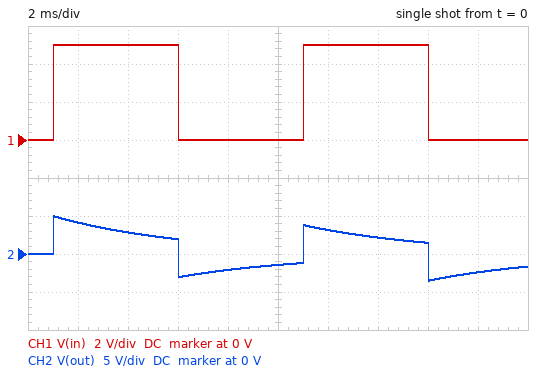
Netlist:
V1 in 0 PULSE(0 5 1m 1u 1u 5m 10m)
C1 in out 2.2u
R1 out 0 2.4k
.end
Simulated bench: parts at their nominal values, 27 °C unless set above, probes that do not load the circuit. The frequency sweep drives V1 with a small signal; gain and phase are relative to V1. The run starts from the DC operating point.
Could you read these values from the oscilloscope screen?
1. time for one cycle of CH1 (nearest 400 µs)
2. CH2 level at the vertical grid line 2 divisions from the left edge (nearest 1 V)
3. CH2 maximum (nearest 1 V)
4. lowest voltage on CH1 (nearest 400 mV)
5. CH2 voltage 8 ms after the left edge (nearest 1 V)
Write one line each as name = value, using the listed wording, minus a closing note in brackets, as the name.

time for one cycle of CH1 = 10.0 ms
CH2 level at the vertical grid line 2 divisions from the left edge = 3 V
CH2 maximum = 5 V
lowest voltage on CH1 = 0 V
CH2 voltage 8 ms after the left edge = -2 V
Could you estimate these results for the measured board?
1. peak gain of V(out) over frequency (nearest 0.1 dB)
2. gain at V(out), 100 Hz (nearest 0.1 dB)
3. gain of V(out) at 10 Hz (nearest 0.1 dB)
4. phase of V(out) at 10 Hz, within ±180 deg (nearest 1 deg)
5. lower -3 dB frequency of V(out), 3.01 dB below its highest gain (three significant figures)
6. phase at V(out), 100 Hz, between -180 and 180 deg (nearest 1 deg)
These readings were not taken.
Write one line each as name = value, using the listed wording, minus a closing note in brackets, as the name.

peak gain of V(out) over frequency = 0 dB
gain at V(out), 100 Hz = -0.4 dB
gain of V(out) at 10 Hz = -10.0 dB
phase of V(out) at 10 Hz, within ±180 deg = 72 deg
lower -3 dB frequency of V(out), 3.01 dB below its highest gain = 30.1 Hz
phase at V(out), 100 Hz, between -180 and 180 deg = 17 deg
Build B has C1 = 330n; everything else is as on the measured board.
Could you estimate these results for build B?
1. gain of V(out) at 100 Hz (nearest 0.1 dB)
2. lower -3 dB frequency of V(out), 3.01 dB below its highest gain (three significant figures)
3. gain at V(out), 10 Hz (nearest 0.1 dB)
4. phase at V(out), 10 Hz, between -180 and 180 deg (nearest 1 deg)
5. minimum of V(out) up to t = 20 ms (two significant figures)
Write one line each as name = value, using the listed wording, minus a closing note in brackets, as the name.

gain of V(out) at 100 Hz = -7.0 dB
lower -3 dB frequency of V(out), 3.01 dB below its highest gain = 201 Hz
gain at V(out), 10 Hz = -26.1 dB
phase at V(out), 10 Hz, between -180 and 180 deg = 87 deg
minimum of V(out) up to t = 20 ms = -5.0 V
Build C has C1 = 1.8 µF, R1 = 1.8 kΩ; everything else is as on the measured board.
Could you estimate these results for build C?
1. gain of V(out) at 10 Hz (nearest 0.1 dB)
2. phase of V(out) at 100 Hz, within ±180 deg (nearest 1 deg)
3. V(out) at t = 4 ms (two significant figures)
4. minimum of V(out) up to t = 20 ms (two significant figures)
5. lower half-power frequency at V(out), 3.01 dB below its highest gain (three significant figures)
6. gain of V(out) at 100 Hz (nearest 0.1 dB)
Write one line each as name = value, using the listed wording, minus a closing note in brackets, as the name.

gain of V(out) at 10 Hz = -14.0 dB
phase of V(out) at 100 Hz, within ±180 deg = 26 deg
V(out) at t = 4 ms = 2.0 V
minimum of V(out) up to t = 20 ms = -4.1 V
lower half-power frequency at V(out), 3.01 dB below its highest gain = 49.1 Hz
gain of V(out) at 100 Hz = -0.9 dB
